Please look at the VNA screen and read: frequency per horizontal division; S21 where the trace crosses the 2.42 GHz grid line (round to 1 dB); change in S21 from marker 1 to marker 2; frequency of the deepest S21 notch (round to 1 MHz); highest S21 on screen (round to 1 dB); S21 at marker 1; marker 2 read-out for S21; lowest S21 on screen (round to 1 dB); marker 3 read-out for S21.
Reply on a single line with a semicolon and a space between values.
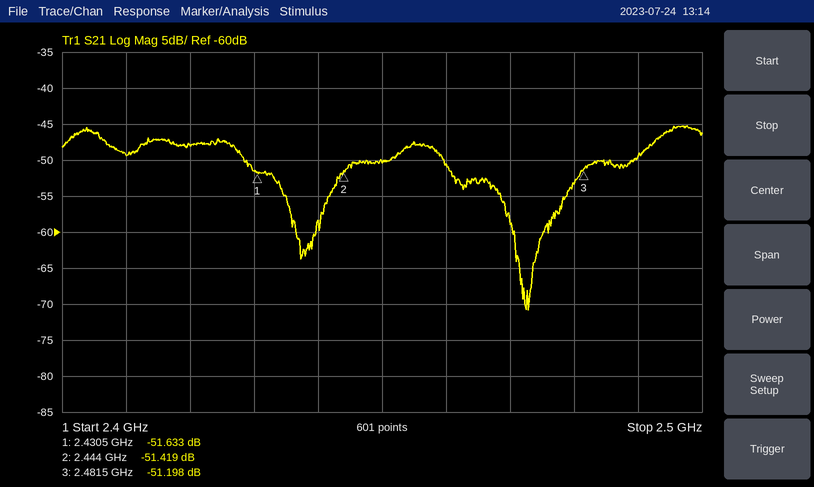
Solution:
10 MHz; -48 dB; 0.214 dB; 2.473 GHz; -45 dB; -51.633 dB; -51.419 dB; -71 dB; -51.198 dB
